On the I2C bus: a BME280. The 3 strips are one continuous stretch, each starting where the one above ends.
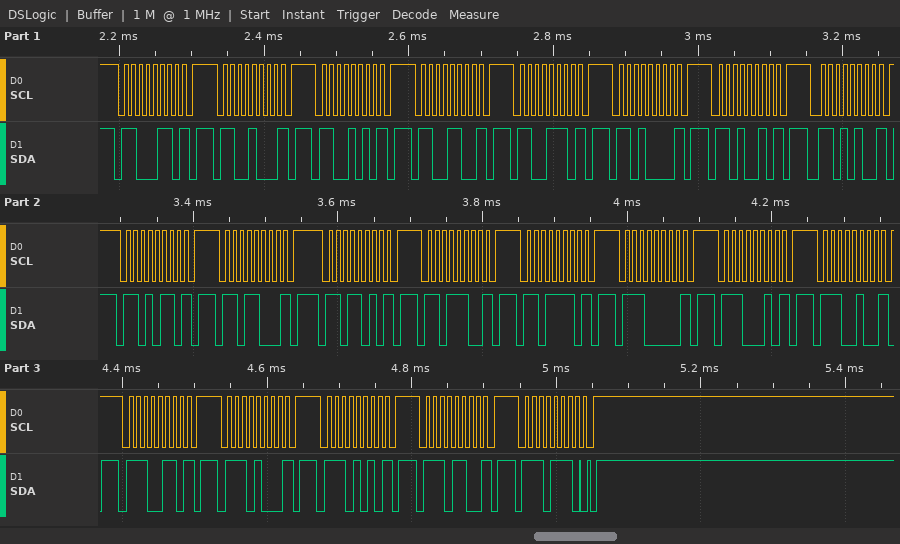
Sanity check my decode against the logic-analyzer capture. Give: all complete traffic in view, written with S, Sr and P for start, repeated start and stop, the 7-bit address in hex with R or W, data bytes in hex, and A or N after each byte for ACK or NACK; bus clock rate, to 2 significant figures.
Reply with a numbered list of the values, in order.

1. S 63W N P S 64W N P S 65W N P S 66W N P S 67W N P S 68W N P S 69W N P S 6AW N P S 6BW N P S 6CW N P S 6DW N P S 6EW N P S 6FW N P S 70W N P S 71W N P S 72W N P S 73W N P S 74W N P S 75W N P S 76W N P S 77W A P
2. 100 kHz
